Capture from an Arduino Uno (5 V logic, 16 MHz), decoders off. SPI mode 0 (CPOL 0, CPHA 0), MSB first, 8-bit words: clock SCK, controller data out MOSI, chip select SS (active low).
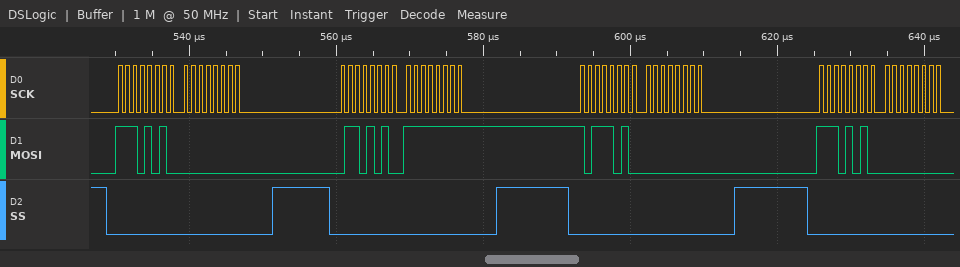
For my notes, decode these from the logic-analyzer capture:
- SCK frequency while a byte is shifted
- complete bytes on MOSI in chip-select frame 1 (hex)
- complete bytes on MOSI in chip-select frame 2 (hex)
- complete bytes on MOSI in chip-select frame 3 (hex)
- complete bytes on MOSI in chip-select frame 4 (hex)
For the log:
1 MHz
EA 00
6A FF
BA 00
EA 00
